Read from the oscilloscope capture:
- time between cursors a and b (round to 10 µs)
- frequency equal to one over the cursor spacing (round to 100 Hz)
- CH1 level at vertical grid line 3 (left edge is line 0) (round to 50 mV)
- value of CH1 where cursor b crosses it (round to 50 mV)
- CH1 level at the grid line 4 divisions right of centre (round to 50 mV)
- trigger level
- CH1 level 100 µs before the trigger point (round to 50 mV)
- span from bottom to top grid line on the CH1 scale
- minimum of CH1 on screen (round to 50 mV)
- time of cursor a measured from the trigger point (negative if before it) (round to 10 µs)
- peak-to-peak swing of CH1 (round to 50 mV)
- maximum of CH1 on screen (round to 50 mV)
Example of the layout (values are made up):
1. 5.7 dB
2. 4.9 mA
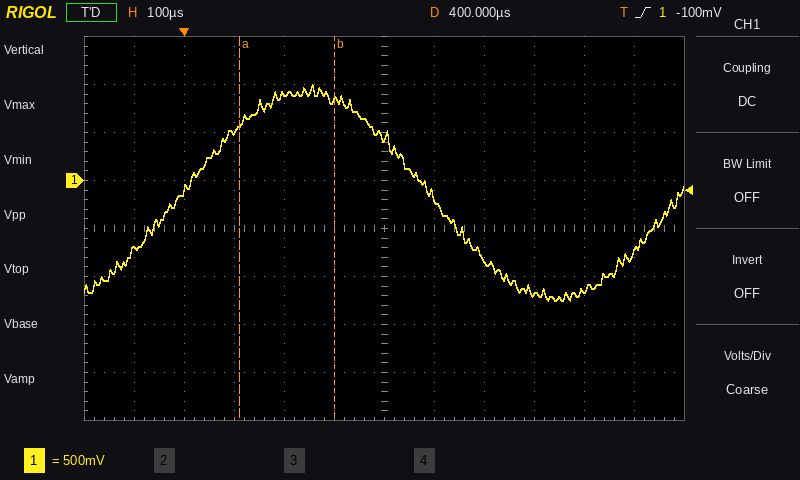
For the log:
1. 190 µs
2. 5.3 kHz
3. 500 mV
4. 850 mV
5. -1.15 V
6. -100 mV
7. -700 mV
8. 4 V
9. -1.25 V
10. +110 µs
11. 2.25 V
12. 1.00 V
